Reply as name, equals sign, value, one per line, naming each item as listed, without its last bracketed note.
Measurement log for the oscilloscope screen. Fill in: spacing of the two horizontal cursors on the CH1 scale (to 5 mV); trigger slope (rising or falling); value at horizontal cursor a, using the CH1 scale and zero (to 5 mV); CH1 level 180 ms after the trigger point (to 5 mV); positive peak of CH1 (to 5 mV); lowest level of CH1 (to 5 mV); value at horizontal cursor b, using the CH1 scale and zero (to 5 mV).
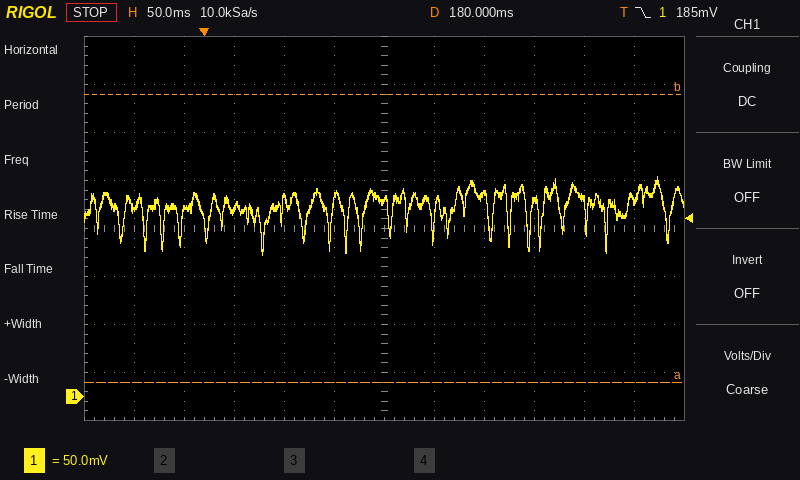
spacing of the two horizontal cursors on the CH1 scale = 300 mV
trigger slope = falling
value at horizontal cursor a, using the CH1 scale and zero = 15 mV
CH1 level 180 ms after the trigger point = 205 mV
positive peak of CH1 = 230 mV
lowest level of CH1 = 145 mV
value at horizontal cursor b, using the CH1 scale and zero = 315 mV
